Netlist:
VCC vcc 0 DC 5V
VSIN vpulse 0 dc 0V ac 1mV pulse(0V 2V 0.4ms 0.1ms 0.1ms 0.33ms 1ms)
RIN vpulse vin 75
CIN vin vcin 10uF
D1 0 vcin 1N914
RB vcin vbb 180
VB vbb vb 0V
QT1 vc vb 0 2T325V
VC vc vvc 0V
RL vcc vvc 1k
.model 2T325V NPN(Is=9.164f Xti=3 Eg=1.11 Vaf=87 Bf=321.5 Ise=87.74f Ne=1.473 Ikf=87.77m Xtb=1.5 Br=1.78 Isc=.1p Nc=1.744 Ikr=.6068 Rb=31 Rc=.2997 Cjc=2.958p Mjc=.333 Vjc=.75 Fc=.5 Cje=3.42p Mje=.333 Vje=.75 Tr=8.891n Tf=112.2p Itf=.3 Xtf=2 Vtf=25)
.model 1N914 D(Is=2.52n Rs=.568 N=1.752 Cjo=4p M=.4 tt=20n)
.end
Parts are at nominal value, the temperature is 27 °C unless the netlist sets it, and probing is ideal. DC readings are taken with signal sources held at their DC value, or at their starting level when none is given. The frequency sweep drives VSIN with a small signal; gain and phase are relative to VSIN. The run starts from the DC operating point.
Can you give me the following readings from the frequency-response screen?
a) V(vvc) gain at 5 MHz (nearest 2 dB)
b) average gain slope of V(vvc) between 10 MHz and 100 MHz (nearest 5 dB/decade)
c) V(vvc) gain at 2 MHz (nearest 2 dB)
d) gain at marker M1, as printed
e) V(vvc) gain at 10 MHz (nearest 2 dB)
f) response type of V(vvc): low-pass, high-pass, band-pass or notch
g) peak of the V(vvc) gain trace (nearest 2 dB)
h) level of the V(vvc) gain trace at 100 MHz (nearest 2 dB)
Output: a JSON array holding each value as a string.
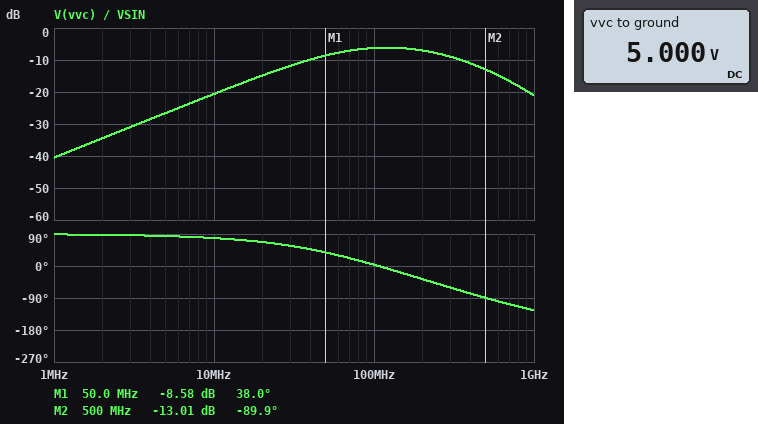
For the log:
["-26 dB", "15 dB/decade", "-34 dB", "-8.58 dB", "-20 dB", "band-pass", "-6 dB", "-6 dB"]
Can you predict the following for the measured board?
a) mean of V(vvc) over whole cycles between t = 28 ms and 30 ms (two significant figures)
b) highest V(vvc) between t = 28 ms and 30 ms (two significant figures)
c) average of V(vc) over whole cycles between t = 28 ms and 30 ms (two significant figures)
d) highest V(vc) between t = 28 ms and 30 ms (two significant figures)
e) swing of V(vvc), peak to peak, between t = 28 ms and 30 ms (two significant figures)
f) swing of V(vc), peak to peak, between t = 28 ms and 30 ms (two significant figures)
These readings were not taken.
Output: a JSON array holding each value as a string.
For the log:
["3.1 V", "5.0 V", "3.1 V", "5.0 V", "5.0 V", "5.0 V"]
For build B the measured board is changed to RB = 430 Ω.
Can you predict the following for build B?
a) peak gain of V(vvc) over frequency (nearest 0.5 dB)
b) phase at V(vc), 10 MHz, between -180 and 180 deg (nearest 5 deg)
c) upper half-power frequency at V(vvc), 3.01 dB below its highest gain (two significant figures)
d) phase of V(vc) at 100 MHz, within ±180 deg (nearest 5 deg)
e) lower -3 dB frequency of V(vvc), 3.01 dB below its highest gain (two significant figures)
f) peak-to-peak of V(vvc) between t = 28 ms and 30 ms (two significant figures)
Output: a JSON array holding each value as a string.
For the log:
["-9.0 dB", "75 deg", "240 MHz", "-10 deg", "33 MHz", "5.0 V"]
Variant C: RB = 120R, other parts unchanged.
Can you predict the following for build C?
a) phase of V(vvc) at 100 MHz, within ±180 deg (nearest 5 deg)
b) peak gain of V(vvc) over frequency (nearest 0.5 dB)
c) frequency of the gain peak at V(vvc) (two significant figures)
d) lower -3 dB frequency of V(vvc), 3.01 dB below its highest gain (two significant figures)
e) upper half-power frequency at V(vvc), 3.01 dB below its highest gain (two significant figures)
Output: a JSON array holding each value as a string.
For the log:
["10 deg", "-5.5 dB", "130 MHz", "49 MHz", "340 MHz"]
